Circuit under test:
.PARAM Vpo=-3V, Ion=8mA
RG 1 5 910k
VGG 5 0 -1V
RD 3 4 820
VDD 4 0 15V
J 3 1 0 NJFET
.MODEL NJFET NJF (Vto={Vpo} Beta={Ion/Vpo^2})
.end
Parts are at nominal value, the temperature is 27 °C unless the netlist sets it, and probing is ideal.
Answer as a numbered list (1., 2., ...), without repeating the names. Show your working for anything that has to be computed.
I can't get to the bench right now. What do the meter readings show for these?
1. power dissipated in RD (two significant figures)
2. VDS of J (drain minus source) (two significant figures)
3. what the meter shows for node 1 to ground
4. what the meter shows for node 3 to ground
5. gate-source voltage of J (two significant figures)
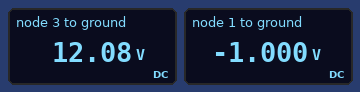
1. (15 V - 12.08 V)^2 / 820 Ω = 10 mW
2. 12.08 V = 12 V
3. -1.000 V
4. 12.08 V
5. -1 V = -1.0 V
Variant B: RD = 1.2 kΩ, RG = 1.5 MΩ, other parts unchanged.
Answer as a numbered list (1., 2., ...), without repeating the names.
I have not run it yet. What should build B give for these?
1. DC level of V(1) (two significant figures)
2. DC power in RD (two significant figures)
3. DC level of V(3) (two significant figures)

1. -1.0 V
2. 15 mW
3. 11 V
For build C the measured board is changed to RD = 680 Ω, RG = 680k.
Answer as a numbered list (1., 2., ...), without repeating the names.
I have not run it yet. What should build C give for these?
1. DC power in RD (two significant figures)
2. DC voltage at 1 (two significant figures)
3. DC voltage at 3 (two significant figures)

1. 8.6 mW
2. -1.0 V
3. 13 V
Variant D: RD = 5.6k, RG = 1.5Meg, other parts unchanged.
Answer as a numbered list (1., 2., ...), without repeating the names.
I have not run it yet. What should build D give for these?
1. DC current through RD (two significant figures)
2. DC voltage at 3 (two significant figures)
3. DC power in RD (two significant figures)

1. 2.5 mA
2. 920 mV
3. 35 mW
